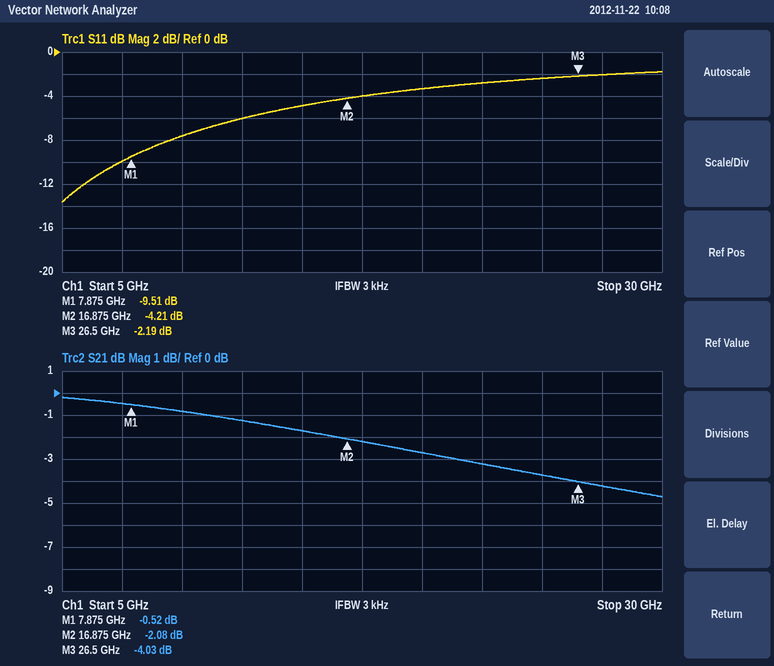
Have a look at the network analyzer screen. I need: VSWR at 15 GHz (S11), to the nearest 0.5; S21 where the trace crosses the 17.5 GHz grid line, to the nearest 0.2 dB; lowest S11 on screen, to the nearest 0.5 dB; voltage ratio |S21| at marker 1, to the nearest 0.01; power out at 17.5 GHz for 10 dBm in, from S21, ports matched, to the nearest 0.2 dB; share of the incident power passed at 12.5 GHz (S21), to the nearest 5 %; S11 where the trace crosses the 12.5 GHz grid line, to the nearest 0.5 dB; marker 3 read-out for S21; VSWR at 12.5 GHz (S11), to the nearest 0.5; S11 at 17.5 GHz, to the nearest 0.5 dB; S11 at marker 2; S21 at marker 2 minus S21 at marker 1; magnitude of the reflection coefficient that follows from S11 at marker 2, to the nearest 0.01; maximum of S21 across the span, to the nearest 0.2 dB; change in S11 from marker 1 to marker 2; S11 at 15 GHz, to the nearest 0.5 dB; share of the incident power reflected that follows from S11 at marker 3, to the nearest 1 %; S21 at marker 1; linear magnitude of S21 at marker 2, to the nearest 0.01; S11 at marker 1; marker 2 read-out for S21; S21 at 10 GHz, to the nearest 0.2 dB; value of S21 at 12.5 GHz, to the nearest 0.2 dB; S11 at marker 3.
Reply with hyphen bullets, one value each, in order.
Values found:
- 3.5
- -2.2 dB
- -13.5 dB
- 0.94
- 7.8 dBm
- 75 %
- -6.0 dB
- -4.03 dB
- 3.0
- -4.0 dB
- -4.21 dB
- -1.56 dB
- 0.62
- -0.2 dB
- 5.30 dB
- -5.0 dB
- 60 %
- -0.52 dB
- 0.79
- -9.51 dB
- -2.08 dB
- -0.8 dB
- -1.2 dB
- -2.19 dB
